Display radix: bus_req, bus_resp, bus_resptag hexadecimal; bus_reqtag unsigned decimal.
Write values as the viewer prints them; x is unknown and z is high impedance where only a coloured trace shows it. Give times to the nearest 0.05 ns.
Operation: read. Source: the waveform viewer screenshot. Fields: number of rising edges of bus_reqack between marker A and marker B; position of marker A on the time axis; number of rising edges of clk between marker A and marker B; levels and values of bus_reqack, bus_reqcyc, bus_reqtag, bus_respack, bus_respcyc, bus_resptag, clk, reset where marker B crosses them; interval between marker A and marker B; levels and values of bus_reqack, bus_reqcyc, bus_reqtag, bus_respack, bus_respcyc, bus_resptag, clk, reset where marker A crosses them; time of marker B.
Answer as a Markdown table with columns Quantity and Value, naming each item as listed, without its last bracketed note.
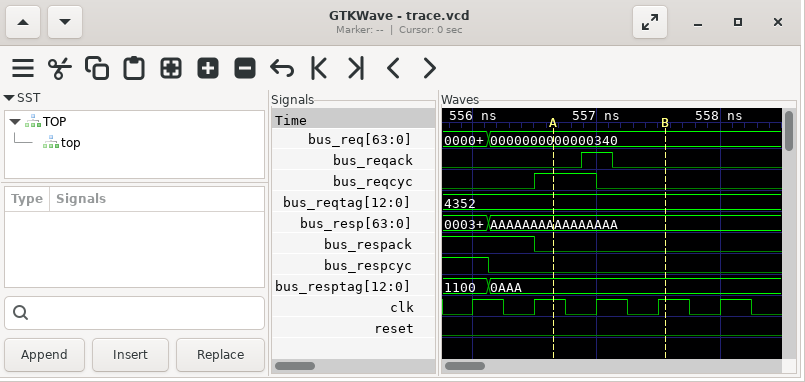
| Quantity | Value |
|---|---|
| number of rising edges of bus_reqack between marker A and marker B | 1 |
| position of marker A on the time axis | 556.65 ns |
| number of rising edges of clk between marker A and marker B | 2 |
| levels and values of bus_reqack, bus_reqcyc, bus_reqtag, bus_respack, bus_respcyc, bus_resptag, clk, reset where marker B crosses them | bus_reqack=0, bus_reqcyc=0, bus_reqtag=4352, bus_respack=0, bus_respcyc=0, bus_resptag=0AAA, clk=1, reset=0 |
| interval between marker A and marker B | 0.9 ns |
| levels and values of bus_reqack, bus_reqcyc, bus_reqtag, bus_respack, bus_respcyc, bus_resptag, clk, reset where marker A crosses them | bus_reqack=0, bus_reqcyc=1, bus_reqtag=4352, bus_respack=0, bus_respcyc=0, bus_resptag=0AAA, clk=1, reset=0 |
| time of marker B | 557.55 ns |
